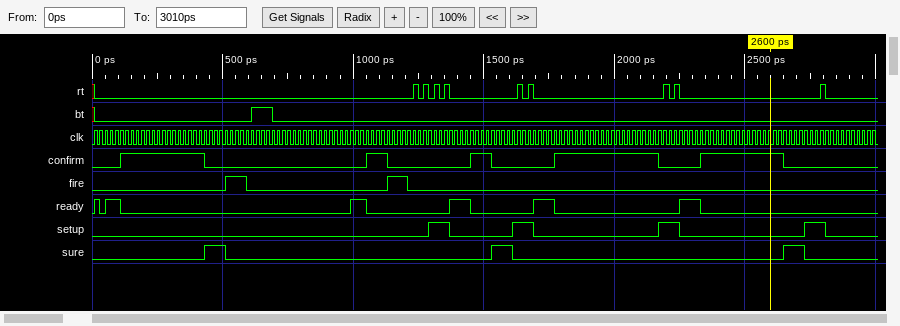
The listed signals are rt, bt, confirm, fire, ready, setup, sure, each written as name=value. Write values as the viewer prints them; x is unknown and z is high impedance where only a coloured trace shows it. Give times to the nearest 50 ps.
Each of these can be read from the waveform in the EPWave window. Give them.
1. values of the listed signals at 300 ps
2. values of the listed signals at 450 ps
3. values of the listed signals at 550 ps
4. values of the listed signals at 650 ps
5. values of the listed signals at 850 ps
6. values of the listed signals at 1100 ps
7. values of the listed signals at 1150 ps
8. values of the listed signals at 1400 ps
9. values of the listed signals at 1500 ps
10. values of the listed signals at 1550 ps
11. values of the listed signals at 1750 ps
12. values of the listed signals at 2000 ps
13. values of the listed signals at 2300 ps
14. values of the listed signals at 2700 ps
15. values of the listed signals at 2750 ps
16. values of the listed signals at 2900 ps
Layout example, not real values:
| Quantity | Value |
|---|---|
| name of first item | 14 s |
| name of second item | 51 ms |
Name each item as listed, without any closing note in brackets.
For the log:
| Quantity | Value |
|---|---|
| values of the listed signals at 300 ps | rt=0, bt=0, confirm=1, fire=0, ready=0, setup=0, sure=0 |
| values of the listed signals at 450 ps | rt=0, bt=0, confirm=0, fire=0, ready=0, setup=0, sure=1 |
| values of the listed signals at 550 ps | rt=0, bt=0, confirm=0, fire=1, ready=0, setup=0, sure=0 |
| values of the listed signals at 650 ps | rt=0, bt=1, confirm=0, fire=0, ready=0, setup=0, sure=0 |
| values of the listed signals at 850 ps | rt=0, bt=0, confirm=0, fire=0, ready=0, setup=0, sure=0 |
| values of the listed signals at 1100 ps | rt=0, bt=0, confirm=1, fire=0, ready=0, setup=0, sure=0 |
| values of the listed signals at 1150 ps | rt=0, bt=0, confirm=0, fire=1, ready=0, setup=0, sure=0 |
| values of the listed signals at 1400 ps | rt=0, bt=0, confirm=0, fire=0, ready=1, setup=0, sure=0 |
| values of the listed signals at 1500 ps | rt=0, bt=0, confirm=1, fire=0, ready=0, setup=0, sure=0 |
| values of the listed signals at 1550 ps | rt=0, bt=0, confirm=0, fire=0, ready=0, setup=0, sure=1 |
| values of the listed signals at 1750 ps | rt=0, bt=0, confirm=0, fire=0, ready=1, setup=0, sure=0 |
| values of the listed signals at 2000 ps | rt=0, bt=0, confirm=1, fire=0, ready=0, setup=0, sure=0 |
| values of the listed signals at 2300 ps | rt=0, bt=0, confirm=0, fire=0, ready=1, setup=0, sure=0 |
| values of the listed signals at 2700 ps | rt=0, bt=0, confirm=0, fire=0, ready=0, setup=0, sure=1 |
| values of the listed signals at 2750 ps | rt=0, bt=0, confirm=0, fire=0, ready=0, setup=1, sure=0 |
| values of the listed signals at 2900 ps | rt=0, bt=0, confirm=0, fire=0, ready=0, setup=0, sure=0 |
